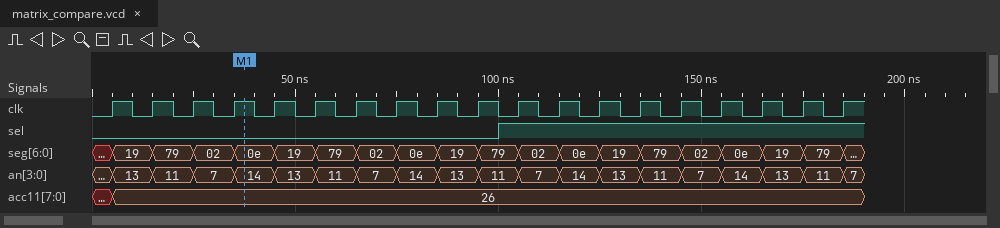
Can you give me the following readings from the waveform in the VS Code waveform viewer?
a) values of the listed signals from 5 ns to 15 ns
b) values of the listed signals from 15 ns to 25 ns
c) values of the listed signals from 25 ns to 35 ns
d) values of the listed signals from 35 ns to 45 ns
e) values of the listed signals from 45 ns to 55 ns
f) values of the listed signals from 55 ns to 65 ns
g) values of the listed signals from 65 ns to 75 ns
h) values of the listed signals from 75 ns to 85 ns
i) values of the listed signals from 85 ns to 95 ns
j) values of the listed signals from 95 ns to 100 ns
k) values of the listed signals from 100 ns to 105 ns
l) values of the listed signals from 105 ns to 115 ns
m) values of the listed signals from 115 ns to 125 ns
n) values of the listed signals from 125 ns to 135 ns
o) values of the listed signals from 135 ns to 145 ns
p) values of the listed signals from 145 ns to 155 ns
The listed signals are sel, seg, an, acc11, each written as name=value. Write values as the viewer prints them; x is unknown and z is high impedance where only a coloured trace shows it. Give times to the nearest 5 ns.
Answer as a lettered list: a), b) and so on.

a) sel=0, seg=19, an=13, acc11=26
b) sel=0, seg=79, an=11, acc11=26
c) sel=0, seg=02, an=7, acc11=26
d) sel=0, seg=0e, an=14, acc11=26
e) sel=0, seg=19, an=13, acc11=26
f) sel=0, seg=79, an=11, acc11=26
g) sel=0, seg=02, an=7, acc11=26
h) sel=0, seg=0e, an=14, acc11=26
i) sel=0, seg=19, an=13, acc11=26
j) sel=0, seg=79, an=11, acc11=26
k) sel=1, seg=79, an=11, acc11=26
l) sel=1, seg=02, an=7, acc11=26
m) sel=1, seg=0e, an=14, acc11=26
n) sel=1, seg=19, an=13, acc11=26
o) sel=1, seg=79, an=11, acc11=26
p) sel=1, seg=02, an=7, acc11=26
